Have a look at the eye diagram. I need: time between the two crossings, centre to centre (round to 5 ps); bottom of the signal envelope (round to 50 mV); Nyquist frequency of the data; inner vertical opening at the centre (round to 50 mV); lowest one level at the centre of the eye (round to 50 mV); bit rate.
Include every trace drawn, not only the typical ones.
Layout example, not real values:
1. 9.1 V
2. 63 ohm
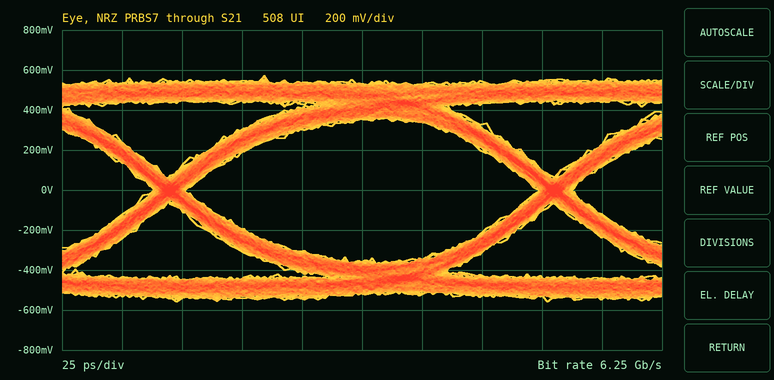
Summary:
1. 160 ps
2. -550 mV
3. 3.125 GHz
4. 700 mV
5. 350 mV
6. 6.25 Gb/s
